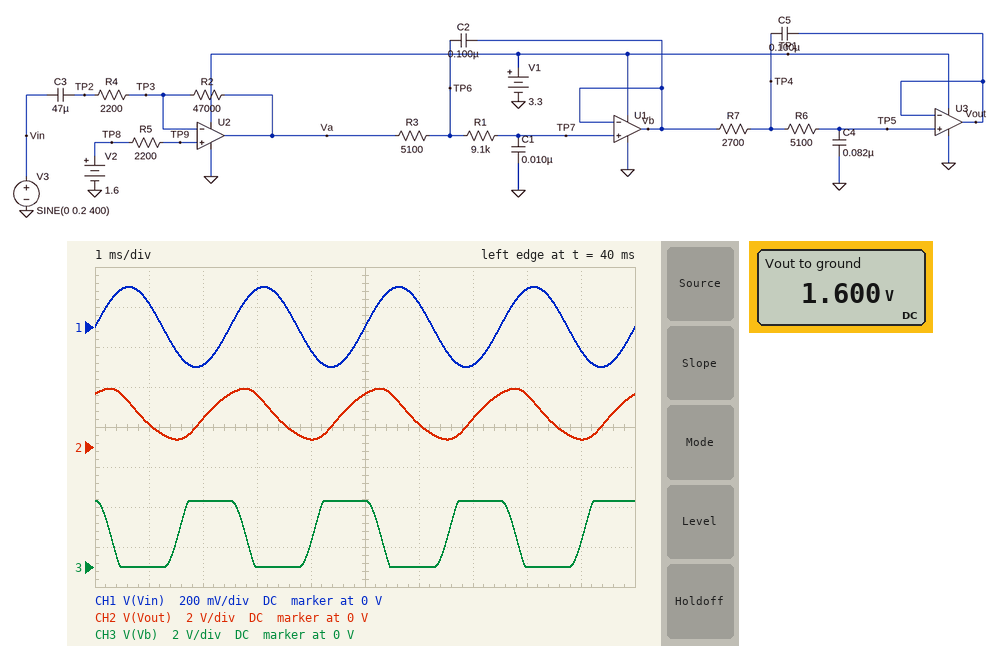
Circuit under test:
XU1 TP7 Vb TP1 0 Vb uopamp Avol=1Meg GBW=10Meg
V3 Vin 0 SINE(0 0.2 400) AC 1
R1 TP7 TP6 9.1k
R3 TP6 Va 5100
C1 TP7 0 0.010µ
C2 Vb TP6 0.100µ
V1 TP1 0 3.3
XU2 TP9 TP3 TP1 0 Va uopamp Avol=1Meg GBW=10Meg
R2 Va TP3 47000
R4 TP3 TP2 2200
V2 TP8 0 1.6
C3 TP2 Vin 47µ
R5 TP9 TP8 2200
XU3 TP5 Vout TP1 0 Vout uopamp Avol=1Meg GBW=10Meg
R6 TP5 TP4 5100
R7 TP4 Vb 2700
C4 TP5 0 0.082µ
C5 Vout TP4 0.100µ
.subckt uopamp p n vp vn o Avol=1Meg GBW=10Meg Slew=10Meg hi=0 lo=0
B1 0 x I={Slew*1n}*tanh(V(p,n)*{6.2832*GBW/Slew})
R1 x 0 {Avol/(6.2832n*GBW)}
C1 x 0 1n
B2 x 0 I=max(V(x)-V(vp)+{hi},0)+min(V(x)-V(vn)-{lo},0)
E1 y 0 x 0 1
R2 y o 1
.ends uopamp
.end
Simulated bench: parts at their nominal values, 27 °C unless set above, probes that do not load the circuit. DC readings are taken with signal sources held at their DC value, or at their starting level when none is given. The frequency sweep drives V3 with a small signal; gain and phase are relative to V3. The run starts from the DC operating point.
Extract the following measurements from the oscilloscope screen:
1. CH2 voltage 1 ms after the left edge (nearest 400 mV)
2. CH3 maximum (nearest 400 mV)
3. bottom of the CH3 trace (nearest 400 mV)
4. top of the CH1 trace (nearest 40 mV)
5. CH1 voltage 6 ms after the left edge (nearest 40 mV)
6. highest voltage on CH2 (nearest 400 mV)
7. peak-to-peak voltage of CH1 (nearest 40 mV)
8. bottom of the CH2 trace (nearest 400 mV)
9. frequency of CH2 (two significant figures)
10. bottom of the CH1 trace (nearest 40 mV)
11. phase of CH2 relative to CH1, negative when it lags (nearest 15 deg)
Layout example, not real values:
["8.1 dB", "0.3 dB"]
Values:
["1.2 V", "3.2 V", "0 V", "200 mV", "120 mV", "2.8 V", "400 mV", "400 mV", "400 Hz", "-200 mV", "60 deg"]
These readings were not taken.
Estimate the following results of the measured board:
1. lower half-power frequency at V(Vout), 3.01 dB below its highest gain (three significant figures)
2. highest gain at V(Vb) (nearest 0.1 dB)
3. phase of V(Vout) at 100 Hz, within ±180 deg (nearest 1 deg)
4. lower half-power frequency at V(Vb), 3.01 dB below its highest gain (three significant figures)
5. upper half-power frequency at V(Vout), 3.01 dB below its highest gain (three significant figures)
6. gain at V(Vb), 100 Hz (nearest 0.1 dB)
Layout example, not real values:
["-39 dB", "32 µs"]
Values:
["1.53 Hz", "30.7 dB", "153 deg", "296 Hz", "505 Hz", "26.7 dB"]
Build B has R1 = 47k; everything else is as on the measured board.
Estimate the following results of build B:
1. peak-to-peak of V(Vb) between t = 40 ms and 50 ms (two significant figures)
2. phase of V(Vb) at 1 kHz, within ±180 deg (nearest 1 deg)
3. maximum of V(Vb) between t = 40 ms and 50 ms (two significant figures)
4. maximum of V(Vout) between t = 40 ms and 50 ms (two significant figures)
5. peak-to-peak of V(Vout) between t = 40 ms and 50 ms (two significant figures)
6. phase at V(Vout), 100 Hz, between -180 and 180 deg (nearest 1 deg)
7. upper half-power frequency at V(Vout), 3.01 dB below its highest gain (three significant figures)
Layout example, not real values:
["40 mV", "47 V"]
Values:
["3.0 V", "21 deg", "3.1 V", "2.5 V", "1.8 V", "138 deg", "312 Hz"]
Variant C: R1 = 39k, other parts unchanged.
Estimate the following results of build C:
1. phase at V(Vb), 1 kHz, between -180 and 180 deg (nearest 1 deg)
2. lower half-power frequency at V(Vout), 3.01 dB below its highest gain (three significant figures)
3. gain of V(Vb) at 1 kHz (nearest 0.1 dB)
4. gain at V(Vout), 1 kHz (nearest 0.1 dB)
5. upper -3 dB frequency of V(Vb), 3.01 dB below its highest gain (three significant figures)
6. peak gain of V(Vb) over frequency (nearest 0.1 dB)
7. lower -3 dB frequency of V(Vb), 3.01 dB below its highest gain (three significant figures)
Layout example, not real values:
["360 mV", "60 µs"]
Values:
["22 deg", "1.55 Hz", "9.2 dB", "-5.3 dB", "418 Hz", "27.9 dB", "2.23 Hz"]
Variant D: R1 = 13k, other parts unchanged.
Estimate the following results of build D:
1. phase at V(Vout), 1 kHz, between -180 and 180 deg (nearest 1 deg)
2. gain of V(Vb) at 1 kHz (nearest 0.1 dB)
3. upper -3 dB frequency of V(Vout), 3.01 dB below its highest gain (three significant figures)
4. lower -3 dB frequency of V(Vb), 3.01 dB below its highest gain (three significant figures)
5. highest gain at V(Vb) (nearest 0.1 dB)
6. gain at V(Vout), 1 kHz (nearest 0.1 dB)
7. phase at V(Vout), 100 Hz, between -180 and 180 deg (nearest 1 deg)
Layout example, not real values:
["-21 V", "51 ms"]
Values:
["-96 deg", "20.7 dB", "532 Hz", "190 Hz", "30.2 dB", "6.2 dB", "151 deg"]
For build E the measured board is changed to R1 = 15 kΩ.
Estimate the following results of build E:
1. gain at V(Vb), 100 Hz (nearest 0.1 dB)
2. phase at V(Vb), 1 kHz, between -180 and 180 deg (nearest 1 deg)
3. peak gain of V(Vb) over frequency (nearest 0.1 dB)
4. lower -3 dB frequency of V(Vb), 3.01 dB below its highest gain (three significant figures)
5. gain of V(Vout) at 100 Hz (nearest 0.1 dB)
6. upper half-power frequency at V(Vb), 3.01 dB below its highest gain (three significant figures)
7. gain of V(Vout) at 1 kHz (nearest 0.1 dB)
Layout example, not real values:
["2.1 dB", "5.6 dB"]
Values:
["26.8 dB", "32 deg", "30.0 dB", "140 Hz", "26.5 dB", "684 Hz", "4.6 dB"]
